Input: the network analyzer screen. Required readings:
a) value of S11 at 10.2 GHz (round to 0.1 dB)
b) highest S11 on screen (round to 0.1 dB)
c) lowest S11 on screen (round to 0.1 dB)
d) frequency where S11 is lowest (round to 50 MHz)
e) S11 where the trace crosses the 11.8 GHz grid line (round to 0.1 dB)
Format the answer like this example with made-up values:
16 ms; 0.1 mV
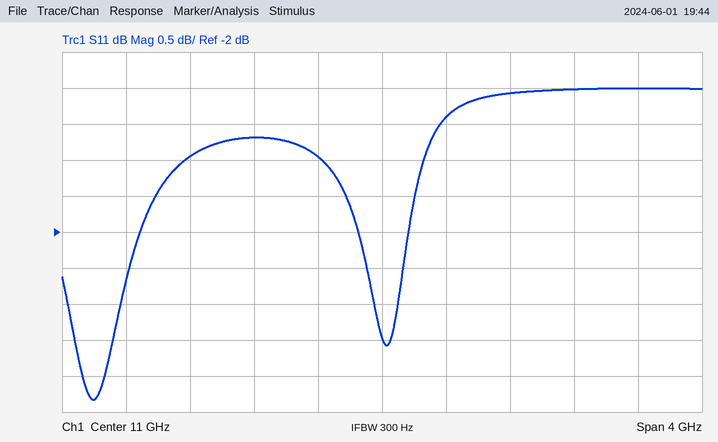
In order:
-0.7 dB; 0.0 dB; -4.3 dB; 9.20 GHz; -0.1 dB
